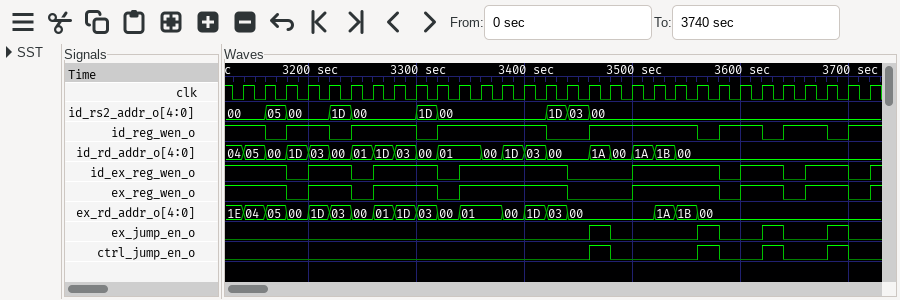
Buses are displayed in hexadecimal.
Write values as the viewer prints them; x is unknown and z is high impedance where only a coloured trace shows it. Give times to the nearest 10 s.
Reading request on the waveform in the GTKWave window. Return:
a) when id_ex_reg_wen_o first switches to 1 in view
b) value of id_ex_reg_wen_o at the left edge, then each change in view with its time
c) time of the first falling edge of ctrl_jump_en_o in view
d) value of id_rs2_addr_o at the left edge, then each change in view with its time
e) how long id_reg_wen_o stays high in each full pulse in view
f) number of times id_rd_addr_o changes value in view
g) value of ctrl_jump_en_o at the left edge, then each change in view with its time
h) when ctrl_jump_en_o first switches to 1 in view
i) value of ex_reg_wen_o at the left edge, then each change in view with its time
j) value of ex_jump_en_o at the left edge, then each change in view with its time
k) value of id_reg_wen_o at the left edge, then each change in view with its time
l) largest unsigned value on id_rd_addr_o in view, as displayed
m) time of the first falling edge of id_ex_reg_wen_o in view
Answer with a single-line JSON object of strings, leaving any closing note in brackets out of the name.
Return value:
{"when id_ex_reg_wen_o first switches to 1 in view": "3200 s", "value of id_ex_reg_wen_o at the left edge, then each change in view with its time": "1, 0 at 3180 s, 1 at 3200 s, 0 at 3240 s, 1 at 3260 s, 0 at 3320 s, 1 at 3340 s, 0 at 3440 s, 1 at 3500 s, 0 at 3580 s, 1 at 3600 s, 0 at 3640 s, 1 at 3660 s, 0 at 3700 s, 1 at 3720 s", "time of the first falling edge of ctrl_jump_en_o in view": "3480 s", "value of id_rs2_addr_o at the left edge, then each change in view with its time": "00, 05 at 3160 s, 00 at 3180 s, 1D at 3220 s, 00 at 3240 s, 1D at 3300 s, 00 at 3320 s, 1D at 3420 s, 03 at 3440 s, 00 at 3460 s", "how long id_reg_wen_o stays high in each full pulse in view": "40 s, 60 s, 100 s, 100 s, 40 s, 40 s", "number of times id_rd_addr_o changes value in view": "19", "value of ctrl_jump_en_o at the left edge, then each change in view with its time": "0, 1 at 3460 s, 0 at 3480 s, 1 at 3560 s, 0 at 3580 s, 1 at 3620 s, 0 at 3640 s, 1 at 3680 s, 0 at 3700 s", "when ctrl_jump_en_o first switches to 1 in view": "3460 s", "value of ex_reg_wen_o at the left edge, then each change in view with its time": "1, 0 at 3180 s, 1 at 3200 s, 0 at 3240 s, 1 at 3260 s, 0 at 3320 s, 1 at 3340 s, 0 at 3440 s, 1 at 3500 s, 0 at 3580 s, 1 at 3600 s, 0 at 3640 s, 1 at 3660 s, 0 at 3700 s, 1 at 3720 s", "value of ex_jump_en_o at the left edge, then each change in view with its time": "0, 1 at 3460 s, 0 at 3480 s, 1 at 3560 s, 0 at 3580 s, 1 at 3620 s, 0 at 3640 s, 1 at 3680 s, 0 at 3700 s", "value of id_reg_wen_o at the left edge, then each change in view with its time": "1, 0 at 3160 s, 1 at 3180 s, 0 at 3220 s, 1 at 3240 s, 0 at 3300 s, 1 at 3320 s, 0 at 3420 s, 1 at 3460 s, 0 at 3560 s, 1 at 3580 s, 0 at 3620 s, 1 at 3640 s, 0 at 3680 s, 1 at 3700 s", "largest unsigned value on id_rd_addr_o in view, as displayed": "1D", "time of the first falling edge of id_ex_reg_wen_o in view": "3180 s"}
